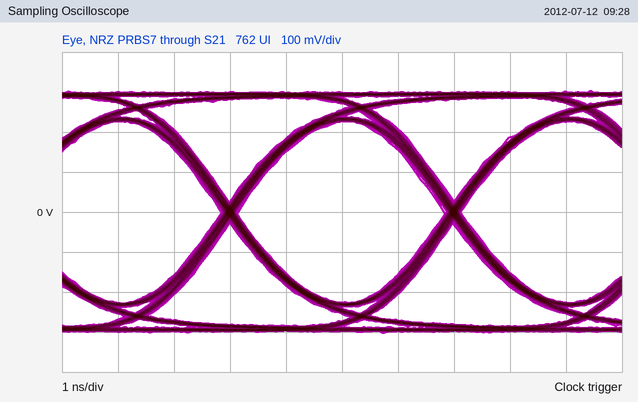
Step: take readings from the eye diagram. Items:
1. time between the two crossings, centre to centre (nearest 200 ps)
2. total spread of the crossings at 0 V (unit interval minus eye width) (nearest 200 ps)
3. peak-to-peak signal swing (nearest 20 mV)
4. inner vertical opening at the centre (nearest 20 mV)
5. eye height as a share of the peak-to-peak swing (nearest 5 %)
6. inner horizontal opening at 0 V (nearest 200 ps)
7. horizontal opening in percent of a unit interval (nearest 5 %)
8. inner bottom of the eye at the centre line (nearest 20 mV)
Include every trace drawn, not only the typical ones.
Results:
4.0 ns
400 ps
600 mV
460 mV
75 %
3.6 ns
90 %
-220 mV
